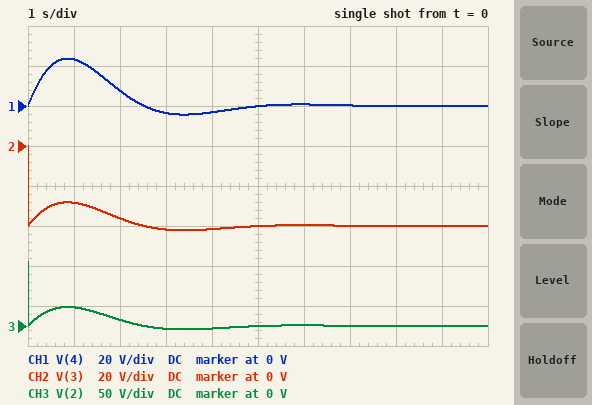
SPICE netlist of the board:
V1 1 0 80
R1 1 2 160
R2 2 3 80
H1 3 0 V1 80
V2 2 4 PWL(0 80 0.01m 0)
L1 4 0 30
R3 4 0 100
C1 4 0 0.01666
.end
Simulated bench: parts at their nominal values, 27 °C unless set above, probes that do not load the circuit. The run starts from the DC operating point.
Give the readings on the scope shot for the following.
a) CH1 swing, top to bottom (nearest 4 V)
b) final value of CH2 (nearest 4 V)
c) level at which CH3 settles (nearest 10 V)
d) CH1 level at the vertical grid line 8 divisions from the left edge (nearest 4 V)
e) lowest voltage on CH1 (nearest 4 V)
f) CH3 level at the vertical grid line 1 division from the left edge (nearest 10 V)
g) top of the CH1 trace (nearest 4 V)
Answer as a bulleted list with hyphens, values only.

- 28 V
- -40 V
- 0 V
- 0 V
- -4 V
- 20 V
- 24 V
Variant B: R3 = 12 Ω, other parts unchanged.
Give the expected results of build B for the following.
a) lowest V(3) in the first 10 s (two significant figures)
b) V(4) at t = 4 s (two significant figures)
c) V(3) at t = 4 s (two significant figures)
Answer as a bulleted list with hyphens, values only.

- -40 V
- 2.7 V
- -39 V
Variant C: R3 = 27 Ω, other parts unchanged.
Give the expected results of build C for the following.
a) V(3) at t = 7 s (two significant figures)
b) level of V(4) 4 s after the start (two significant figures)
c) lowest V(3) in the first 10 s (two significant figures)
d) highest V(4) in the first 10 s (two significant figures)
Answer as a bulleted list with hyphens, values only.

- -40 V
- 1.0 V
- -40 V
- 15 V
